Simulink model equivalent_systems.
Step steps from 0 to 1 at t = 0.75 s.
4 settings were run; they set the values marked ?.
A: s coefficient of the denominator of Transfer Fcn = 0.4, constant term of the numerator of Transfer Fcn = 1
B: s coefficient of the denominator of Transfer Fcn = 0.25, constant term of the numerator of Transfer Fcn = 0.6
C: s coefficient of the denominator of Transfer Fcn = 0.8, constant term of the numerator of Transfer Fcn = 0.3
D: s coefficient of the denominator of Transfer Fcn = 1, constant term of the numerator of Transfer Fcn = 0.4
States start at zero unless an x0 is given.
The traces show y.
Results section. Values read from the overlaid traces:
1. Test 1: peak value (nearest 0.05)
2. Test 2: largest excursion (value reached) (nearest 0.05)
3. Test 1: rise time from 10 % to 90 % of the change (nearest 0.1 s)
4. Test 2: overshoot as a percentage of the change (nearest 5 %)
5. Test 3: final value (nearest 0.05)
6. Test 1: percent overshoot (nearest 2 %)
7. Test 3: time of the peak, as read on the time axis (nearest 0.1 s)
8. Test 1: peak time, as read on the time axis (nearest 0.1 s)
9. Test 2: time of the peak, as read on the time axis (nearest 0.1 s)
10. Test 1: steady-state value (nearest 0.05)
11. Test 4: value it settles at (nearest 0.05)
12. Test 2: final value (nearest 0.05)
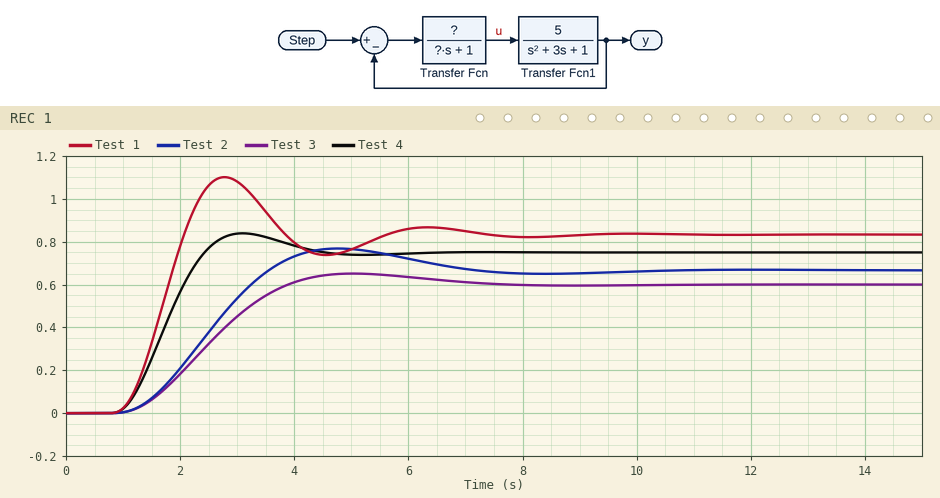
1.10
0.75
0.8 s
15 %
0.60
32 %
5.0 s
2.8 s
4.8 s
0.85
0.75
0.65
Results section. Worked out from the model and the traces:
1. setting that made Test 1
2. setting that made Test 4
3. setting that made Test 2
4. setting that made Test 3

A
B
D
C
